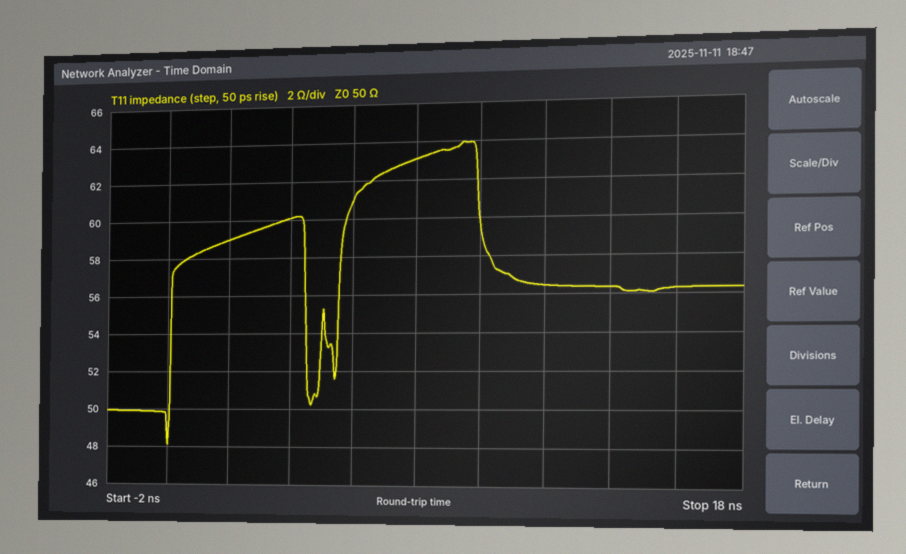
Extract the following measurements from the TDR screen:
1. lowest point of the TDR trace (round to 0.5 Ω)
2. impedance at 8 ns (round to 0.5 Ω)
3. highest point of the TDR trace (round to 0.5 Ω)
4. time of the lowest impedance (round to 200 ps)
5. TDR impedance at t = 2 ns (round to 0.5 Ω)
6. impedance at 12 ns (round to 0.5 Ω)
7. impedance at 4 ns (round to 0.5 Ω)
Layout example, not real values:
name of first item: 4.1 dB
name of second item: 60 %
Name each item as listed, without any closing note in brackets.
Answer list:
lowest point of the TDR trace: 48.0 Ω
impedance at 8 ns: 63.0 Ω
highest point of the TDR trace: 64.0 Ω
time of the lowest impedance: 0.0 ns
TDR impedance at t = 2 ns: 59.0 Ω
impedance at 12 ns: 56.5 Ω
impedance at 4 ns: 60.0 Ω
